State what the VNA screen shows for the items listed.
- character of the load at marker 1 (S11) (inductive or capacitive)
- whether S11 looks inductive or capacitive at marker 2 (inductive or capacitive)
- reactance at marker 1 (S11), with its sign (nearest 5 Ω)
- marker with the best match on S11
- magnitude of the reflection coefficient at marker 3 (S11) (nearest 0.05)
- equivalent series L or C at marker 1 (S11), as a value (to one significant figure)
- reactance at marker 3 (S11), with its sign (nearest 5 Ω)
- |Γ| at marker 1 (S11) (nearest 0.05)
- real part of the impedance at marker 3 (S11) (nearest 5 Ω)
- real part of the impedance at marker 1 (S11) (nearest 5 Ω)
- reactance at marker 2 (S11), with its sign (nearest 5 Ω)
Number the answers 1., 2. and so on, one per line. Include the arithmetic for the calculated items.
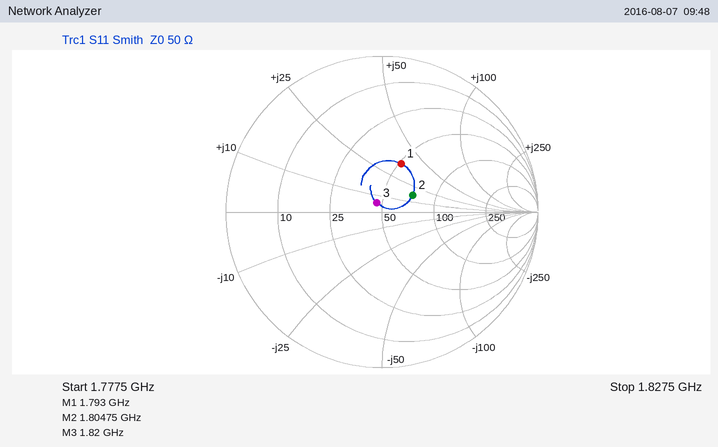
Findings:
1. inductive
2. inductive
3. +35 Ω
4. marker 3
5. 0.05
6. L = 35 Ω/(2π × 1.793 GHz) ≈ 3 nH
7. +5 Ω
8. 0.35
9. 45 Ω
10. 50 Ω
11. +15 Ω
